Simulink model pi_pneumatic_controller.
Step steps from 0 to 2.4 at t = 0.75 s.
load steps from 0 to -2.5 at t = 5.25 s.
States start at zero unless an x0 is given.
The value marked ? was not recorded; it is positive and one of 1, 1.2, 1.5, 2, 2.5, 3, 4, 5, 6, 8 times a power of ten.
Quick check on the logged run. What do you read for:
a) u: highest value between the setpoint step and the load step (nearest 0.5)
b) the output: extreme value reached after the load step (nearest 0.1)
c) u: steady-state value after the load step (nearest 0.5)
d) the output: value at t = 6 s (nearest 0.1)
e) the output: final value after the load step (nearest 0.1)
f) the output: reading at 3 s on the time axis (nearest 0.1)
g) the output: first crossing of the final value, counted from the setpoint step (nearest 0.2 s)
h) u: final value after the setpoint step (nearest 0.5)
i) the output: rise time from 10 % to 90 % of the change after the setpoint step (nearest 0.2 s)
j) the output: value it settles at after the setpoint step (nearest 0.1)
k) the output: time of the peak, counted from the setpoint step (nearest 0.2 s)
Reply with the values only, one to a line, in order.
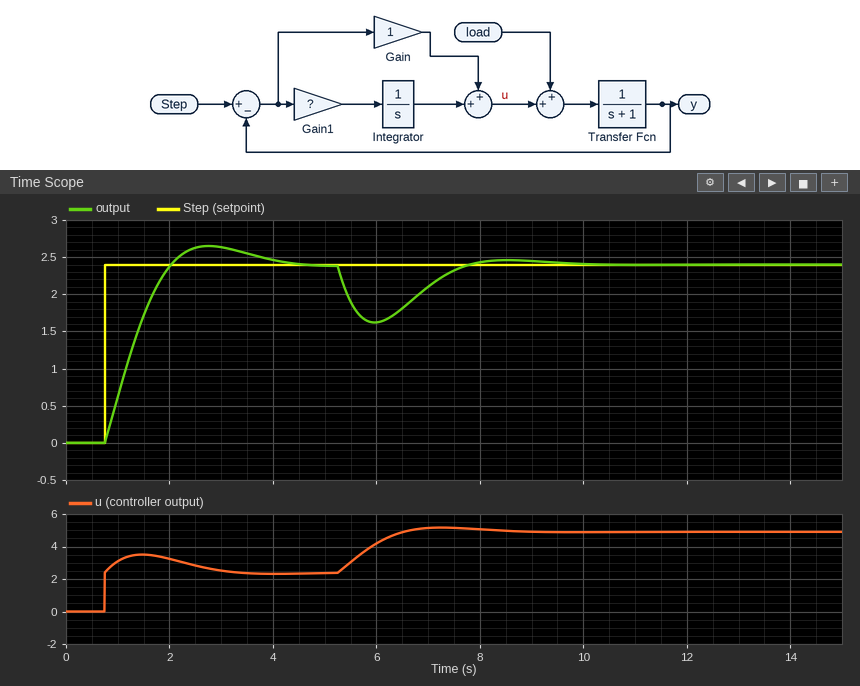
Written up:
3.5
1.6
5.0
1.6
2.4
2.6
1.2 s
2.5
1.0 s
2.4
2.0 s
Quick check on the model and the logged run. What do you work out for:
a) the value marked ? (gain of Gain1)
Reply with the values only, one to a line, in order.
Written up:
2.5
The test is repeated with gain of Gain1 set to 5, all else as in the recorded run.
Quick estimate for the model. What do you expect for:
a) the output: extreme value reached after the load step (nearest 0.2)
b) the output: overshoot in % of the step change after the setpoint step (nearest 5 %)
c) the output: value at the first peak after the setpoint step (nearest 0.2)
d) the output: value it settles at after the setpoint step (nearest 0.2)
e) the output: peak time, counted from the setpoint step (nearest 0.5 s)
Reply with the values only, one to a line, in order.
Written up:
1.8
25 %
3.0
2.4
1.5 s
